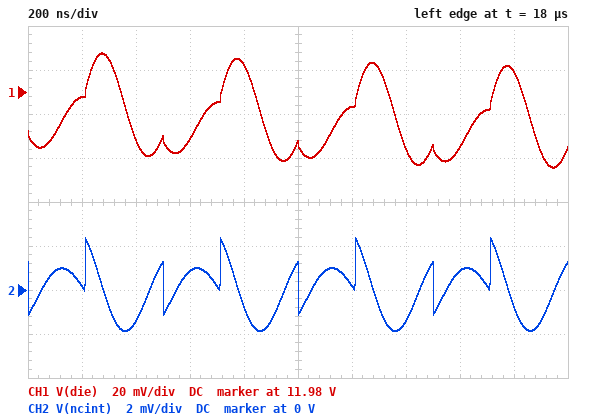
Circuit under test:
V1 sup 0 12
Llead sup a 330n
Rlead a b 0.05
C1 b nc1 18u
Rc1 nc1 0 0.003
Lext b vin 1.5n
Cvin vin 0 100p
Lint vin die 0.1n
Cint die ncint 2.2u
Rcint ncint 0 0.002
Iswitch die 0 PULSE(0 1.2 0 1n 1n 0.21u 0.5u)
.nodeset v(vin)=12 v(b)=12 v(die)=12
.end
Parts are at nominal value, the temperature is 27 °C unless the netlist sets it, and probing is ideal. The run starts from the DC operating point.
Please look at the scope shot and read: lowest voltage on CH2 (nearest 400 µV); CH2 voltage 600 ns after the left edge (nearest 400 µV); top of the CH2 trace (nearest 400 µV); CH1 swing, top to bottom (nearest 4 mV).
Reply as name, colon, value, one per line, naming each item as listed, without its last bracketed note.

lowest voltage on CH2: -2.0 mV
CH2 voltage 600 ns after the left edge: 800 µV
top of the CH2 trace: 2.4 mV
CH1 swing, top to bottom: 52 mV
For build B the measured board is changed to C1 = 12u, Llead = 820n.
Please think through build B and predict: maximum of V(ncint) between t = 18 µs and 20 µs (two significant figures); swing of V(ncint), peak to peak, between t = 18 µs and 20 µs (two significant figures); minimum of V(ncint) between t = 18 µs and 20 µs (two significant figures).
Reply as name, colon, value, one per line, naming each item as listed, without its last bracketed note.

maximum of V(ncint) between t = 18 µs and 20 µs: 2.2 mV
swing of V(ncint), peak to peak, between t = 18 µs and 20 µs: 3.9 mV
minimum of V(ncint) between t = 18 µs and 20 µs: -1.7 mV
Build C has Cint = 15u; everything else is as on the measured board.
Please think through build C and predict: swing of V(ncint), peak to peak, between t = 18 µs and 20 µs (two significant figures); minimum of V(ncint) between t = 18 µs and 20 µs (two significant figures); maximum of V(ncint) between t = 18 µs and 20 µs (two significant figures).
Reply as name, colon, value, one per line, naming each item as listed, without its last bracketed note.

swing of V(ncint), peak to peak, between t = 18 µs and 20 µs: 3.9 mV
minimum of V(ncint) between t = 18 µs and 20 µs: -2.2 mV
maximum of V(ncint) between t = 18 µs and 20 µs: 1.7 mV
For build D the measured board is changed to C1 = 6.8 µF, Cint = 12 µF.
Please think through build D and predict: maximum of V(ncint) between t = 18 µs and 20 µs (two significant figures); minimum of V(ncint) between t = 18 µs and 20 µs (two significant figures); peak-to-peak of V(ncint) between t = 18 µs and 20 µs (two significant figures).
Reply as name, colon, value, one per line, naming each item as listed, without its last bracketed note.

maximum of V(ncint) between t = 18 µs and 20 µs: 3.0 mV
minimum of V(ncint) between t = 18 µs and 20 µs: -3.4 mV
peak-to-peak of V(ncint) between t = 18 µs and 20 µs: 6.4 mV
